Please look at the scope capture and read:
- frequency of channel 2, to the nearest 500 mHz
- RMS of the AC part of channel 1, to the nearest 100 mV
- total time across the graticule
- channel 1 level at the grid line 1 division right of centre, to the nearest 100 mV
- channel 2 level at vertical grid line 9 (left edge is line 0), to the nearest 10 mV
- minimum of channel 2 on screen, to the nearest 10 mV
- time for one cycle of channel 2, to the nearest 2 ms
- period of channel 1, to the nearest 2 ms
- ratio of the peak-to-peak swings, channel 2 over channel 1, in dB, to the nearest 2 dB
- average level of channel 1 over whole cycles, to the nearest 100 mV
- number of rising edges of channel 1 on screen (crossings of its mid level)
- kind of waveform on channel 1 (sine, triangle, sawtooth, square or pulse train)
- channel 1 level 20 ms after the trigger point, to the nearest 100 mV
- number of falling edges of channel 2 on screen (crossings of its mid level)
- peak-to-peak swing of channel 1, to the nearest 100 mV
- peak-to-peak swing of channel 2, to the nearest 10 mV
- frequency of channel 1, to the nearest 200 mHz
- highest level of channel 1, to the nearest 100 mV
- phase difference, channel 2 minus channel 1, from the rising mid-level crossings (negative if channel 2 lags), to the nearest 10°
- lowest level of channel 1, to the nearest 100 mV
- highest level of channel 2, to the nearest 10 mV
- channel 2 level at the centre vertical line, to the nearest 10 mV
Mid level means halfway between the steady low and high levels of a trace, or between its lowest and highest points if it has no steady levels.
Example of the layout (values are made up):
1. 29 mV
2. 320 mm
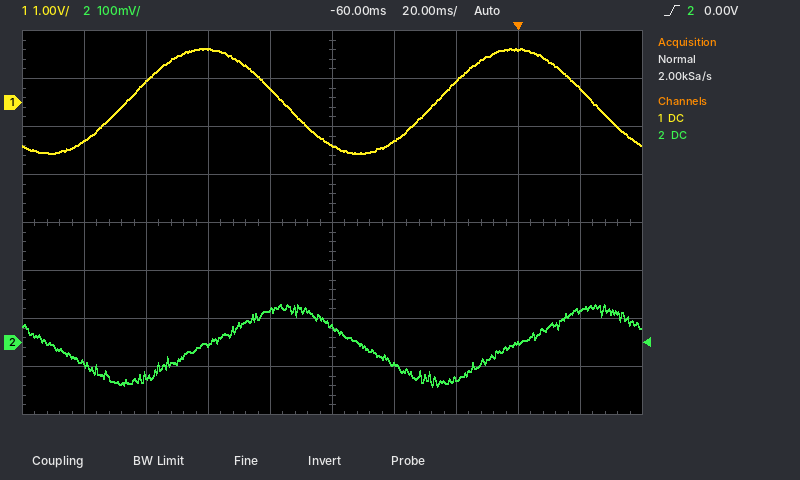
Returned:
1. 10.0 Hz
2. 800 mV
3. 200 ms
4. -800 mV
5. 70 mV
6. -90 mV
7. 100 ms
8. 100 ms
9. -22 dB
10. 0.0 V
11. 2
12. sine
13. 300 mV
14. 2
15. 2.2 V
16. 170 mV
17. 10.0 Hz
18. 1.1 V
19. -90°
20. -1.1 V
21. 80 mV
22. 30 mV
